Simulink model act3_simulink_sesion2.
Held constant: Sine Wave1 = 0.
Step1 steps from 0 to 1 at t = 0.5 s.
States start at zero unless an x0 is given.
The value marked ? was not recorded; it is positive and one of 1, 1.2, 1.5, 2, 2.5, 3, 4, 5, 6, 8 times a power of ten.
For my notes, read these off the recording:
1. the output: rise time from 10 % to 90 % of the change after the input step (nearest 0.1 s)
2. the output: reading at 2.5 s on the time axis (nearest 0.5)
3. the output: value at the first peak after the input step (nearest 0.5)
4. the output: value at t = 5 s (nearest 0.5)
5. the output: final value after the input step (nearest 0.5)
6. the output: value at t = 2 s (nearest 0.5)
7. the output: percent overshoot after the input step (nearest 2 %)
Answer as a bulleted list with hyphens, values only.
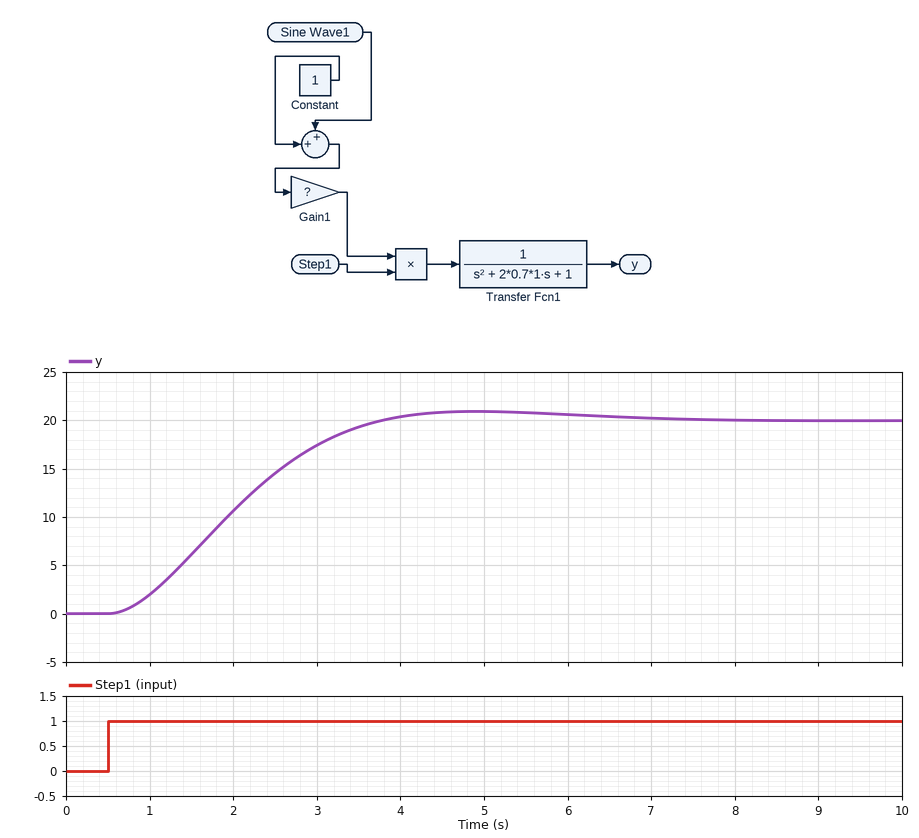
- 2.1 s
- 14.5
- 21.0
- 21.0
- 20.0
- 10.5
- 4 %
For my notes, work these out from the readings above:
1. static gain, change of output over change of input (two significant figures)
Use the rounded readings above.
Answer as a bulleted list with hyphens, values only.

- 20
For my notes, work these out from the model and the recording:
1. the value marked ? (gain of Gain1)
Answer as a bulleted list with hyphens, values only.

- 20
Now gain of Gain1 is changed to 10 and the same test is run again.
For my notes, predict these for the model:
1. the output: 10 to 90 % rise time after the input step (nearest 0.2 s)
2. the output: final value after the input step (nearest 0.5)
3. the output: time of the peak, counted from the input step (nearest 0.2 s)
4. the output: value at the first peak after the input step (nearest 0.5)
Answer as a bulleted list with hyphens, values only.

- 2.2 s
- 10.0
- 4.4 s
- 10.5
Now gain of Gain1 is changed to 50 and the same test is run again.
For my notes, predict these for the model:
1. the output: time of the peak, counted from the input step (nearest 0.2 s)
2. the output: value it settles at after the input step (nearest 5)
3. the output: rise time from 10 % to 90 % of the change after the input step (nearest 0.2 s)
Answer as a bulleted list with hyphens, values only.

- 4.4 s
- 50
- 2.2 s
